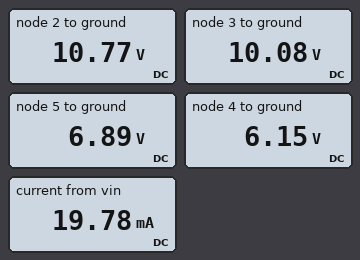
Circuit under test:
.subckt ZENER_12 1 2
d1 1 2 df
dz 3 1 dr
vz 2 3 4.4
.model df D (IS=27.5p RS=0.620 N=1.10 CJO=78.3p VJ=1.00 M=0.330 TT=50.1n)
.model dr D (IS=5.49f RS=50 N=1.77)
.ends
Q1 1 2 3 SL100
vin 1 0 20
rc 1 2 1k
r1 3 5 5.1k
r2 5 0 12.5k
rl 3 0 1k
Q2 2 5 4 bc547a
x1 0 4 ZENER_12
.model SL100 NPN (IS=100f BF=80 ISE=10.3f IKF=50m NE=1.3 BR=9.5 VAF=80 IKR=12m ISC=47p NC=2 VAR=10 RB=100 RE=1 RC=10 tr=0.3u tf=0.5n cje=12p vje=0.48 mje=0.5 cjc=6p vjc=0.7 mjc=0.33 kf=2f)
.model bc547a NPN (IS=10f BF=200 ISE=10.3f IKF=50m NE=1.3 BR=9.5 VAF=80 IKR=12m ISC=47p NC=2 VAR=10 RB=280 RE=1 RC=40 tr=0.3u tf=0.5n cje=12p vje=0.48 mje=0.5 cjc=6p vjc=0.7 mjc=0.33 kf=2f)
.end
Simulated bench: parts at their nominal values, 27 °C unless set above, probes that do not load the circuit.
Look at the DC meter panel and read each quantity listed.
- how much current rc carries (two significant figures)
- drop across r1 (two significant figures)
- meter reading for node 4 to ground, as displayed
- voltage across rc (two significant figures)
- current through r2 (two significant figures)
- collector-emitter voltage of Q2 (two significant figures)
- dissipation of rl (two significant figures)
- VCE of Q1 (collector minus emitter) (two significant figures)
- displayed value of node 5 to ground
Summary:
9.2 mA
3.2 V
6.15 V
9.2 V
550 µA
4.6 V
100 mW
9.9 V
6.89 V
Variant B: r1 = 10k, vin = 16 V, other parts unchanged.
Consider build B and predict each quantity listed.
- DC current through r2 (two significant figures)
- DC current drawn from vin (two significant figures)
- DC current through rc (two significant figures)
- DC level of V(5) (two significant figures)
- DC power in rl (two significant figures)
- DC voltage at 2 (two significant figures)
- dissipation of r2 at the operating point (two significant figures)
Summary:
520 µA
16 mA
3.4 mA
6.5 V
140 mW
13 V
3.4 mW
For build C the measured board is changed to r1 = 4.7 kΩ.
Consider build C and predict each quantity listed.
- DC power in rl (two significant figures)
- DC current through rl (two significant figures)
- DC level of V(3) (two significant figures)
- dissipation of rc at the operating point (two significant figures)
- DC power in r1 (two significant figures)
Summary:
97 mW
9.9 mA
9.9 V
89 mW
1.9 mW
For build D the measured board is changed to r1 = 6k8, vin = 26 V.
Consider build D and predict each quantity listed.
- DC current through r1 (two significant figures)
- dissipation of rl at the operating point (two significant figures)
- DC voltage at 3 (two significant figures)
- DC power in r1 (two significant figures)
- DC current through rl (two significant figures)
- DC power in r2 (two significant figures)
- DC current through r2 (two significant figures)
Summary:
680 µA
140 mW
12 V
3.2 mW
12 mA
4.1 mW
570 µA
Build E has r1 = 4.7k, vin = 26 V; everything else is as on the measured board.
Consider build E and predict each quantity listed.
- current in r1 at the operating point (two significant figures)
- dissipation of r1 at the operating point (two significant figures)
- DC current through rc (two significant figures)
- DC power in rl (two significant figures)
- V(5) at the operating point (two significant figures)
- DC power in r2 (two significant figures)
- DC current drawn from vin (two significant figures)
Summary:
710 µA
2.3 mW
15 mA
110 mW
7.2 V
4.2 mW
26 mA
